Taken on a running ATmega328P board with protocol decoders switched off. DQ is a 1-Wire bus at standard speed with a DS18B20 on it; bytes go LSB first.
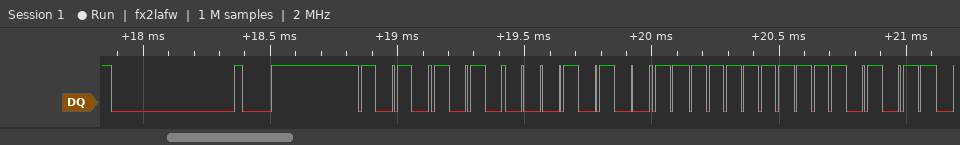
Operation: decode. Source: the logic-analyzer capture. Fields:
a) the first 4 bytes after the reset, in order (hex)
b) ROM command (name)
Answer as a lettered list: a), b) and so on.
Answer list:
a) 55 28 FF D7
b) Match ROM
